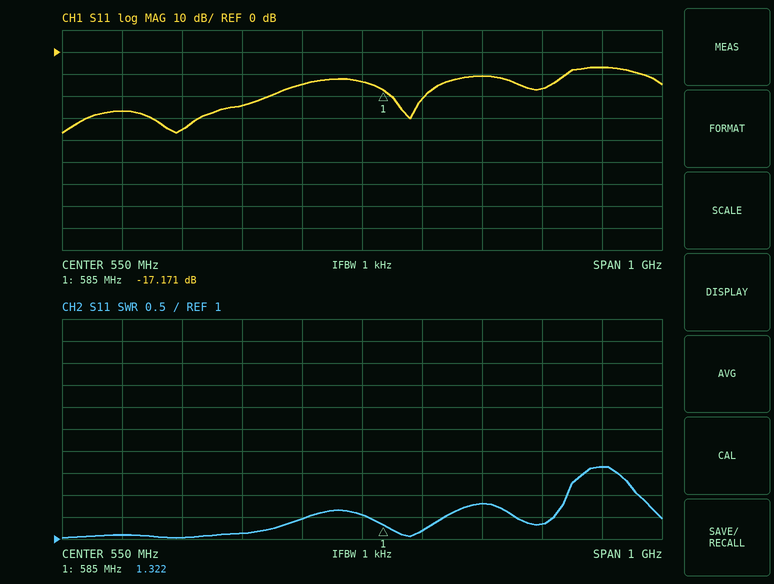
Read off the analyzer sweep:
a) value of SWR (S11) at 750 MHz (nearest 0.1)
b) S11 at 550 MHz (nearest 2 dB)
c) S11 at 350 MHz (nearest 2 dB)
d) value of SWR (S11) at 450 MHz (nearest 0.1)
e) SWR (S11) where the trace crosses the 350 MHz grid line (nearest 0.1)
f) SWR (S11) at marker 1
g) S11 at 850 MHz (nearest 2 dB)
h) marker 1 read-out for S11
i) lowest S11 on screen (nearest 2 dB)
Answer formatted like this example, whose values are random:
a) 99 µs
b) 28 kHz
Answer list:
a) 1.8
b) -14 dB
c) -24 dB
d) 1.5
e) 1.1
f) 1.322
g) -16 dB
h) -17.171 dB
i) -36 dB
